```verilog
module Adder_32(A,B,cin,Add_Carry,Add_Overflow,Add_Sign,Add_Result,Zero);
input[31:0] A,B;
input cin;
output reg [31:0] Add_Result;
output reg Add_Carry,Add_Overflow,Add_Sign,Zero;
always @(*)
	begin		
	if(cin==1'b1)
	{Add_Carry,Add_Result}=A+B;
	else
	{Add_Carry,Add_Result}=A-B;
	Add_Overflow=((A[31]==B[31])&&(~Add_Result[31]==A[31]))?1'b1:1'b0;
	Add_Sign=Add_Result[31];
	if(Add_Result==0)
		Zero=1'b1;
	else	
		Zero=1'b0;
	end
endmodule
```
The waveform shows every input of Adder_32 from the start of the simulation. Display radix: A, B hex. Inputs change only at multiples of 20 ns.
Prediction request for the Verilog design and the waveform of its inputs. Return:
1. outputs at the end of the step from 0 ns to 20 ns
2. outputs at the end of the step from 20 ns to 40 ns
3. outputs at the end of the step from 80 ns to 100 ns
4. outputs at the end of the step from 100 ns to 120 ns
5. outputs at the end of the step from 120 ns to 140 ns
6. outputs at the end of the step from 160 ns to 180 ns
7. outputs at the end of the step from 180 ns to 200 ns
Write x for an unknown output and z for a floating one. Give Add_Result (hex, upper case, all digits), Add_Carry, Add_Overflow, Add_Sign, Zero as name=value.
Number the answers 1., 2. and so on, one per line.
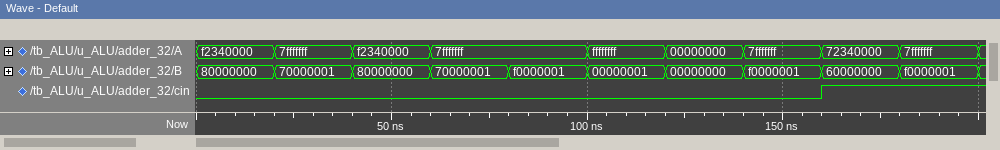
1. Add_Result=72340000, Add_Carry=0, Add_Overflow=1, Add_Sign=0, Zero=0
2. Add_Result=0FFFFFFE, Add_Carry=0, Add_Overflow=0, Add_Sign=0, Zero=0
3. Add_Result=8FFFFFFE, Add_Carry=1, Add_Overflow=0, Add_Sign=1, Zero=0
4. Add_Result=FFFFFFFE, Add_Carry=0, Add_Overflow=0, Add_Sign=1, Zero=0
5. Add_Result=00000000, Add_Carry=0, Add_Overflow=0, Add_Sign=0, Zero=1
6. Add_Result=D2340000, Add_Carry=0, Add_Overflow=1, Add_Sign=1, Zero=0
7. Add_Result=70000000, Add_Carry=1, Add_Overflow=0, Add_Sign=0, Zero=0
